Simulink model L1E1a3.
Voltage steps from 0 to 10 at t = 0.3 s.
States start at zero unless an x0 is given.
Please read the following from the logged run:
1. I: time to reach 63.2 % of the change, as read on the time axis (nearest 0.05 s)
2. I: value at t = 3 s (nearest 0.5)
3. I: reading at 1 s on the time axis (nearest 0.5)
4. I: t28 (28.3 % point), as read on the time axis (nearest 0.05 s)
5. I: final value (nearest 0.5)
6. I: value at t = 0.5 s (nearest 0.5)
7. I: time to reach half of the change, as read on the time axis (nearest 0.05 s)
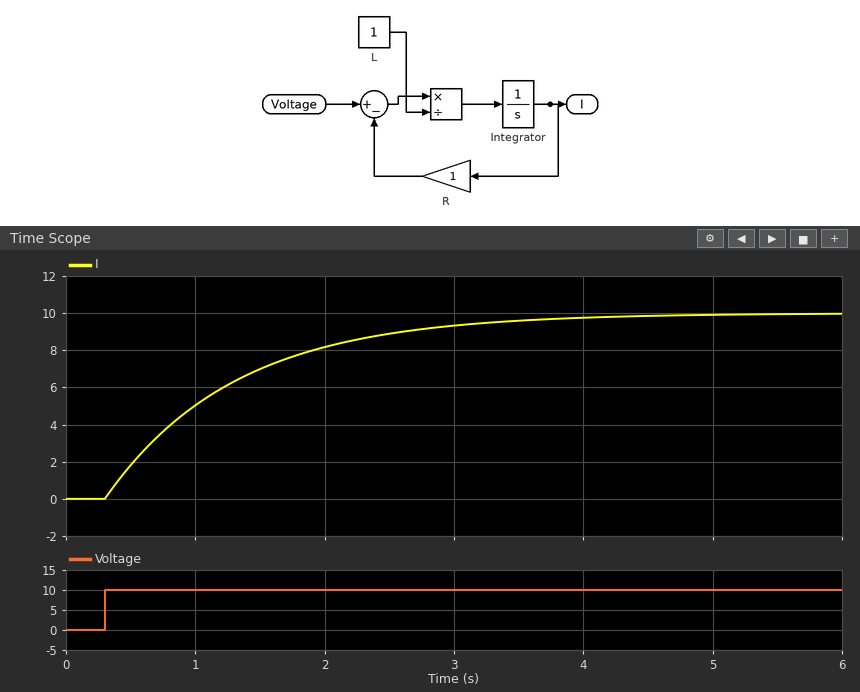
1.30 s
9.5
5.0
0.65 s
10.0
2.0
1.00 s
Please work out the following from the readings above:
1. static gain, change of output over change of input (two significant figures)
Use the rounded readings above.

1.0
